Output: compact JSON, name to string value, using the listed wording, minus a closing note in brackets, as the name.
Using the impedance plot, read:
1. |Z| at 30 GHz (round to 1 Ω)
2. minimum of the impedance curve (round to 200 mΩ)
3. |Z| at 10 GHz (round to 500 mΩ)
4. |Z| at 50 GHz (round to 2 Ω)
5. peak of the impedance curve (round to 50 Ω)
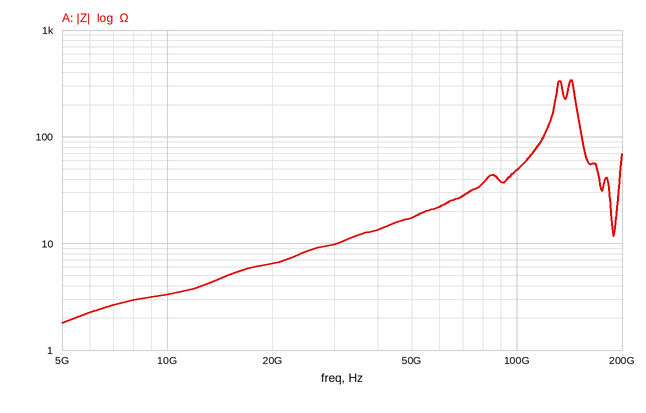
{"|Z| at 30 GHz": "10 Ω", "minimum of the impedance curve": "1.8 Ω", "|Z| at 10 GHz": "3.5 Ω", "|Z| at 50 GHz": "18 Ω", "peak of the impedance curve": "350 Ω"}
